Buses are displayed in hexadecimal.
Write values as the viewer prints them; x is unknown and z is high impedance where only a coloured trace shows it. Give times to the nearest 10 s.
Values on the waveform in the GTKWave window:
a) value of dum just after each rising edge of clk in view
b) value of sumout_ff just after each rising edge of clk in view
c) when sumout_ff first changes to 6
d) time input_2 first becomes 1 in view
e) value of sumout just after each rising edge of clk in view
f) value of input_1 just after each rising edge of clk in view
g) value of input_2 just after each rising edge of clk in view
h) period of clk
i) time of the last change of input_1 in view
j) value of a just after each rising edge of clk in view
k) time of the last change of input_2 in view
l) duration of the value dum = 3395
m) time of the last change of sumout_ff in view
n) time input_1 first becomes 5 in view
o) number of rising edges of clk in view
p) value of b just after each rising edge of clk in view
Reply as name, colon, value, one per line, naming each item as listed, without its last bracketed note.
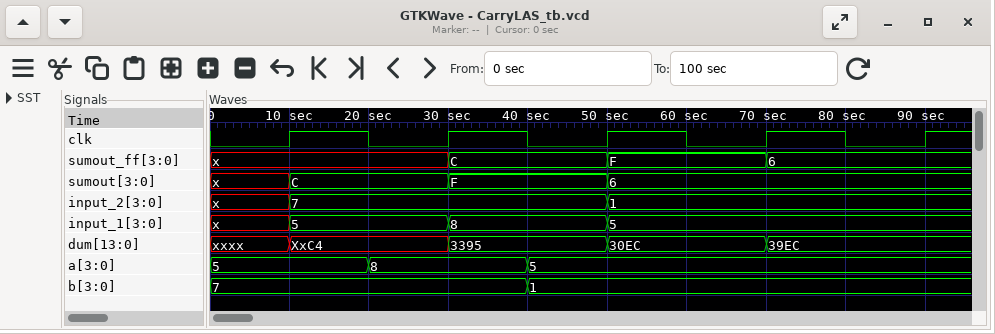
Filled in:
value of dum just after each rising edge of clk in view: XxC4, 3395, 30EC, 39EC, 39EC
value of sumout_ff just after each rising edge of clk in view: x, C, F, 6, 6
when sumout_ff first changes to 6: 70 s
time input_2 first becomes 1 in view: 50 s
value of sumout just after each rising edge of clk in view: C, F, 6, 6, 6
value of input_1 just after each rising edge of clk in view: 5, 8, 5, 5, 5
value of input_2 just after each rising edge of clk in view: 7, 7, 1, 1, 1
period of clk: 20 s
time of the last change of input_1 in view: 50 s
value of a just after each rising edge of clk in view: 5, 8, 5, 5, 5
time of the last change of input_2 in view: 50 s
duration of the value dum = 3395: 20 s
time of the last change of sumout_ff in view: 70 s
time input_1 first becomes 5 in view: 10 s
number of rising edges of clk in view: 5
value of b just after each rising edge of clk in view: 7, 7, 1, 1, 1
